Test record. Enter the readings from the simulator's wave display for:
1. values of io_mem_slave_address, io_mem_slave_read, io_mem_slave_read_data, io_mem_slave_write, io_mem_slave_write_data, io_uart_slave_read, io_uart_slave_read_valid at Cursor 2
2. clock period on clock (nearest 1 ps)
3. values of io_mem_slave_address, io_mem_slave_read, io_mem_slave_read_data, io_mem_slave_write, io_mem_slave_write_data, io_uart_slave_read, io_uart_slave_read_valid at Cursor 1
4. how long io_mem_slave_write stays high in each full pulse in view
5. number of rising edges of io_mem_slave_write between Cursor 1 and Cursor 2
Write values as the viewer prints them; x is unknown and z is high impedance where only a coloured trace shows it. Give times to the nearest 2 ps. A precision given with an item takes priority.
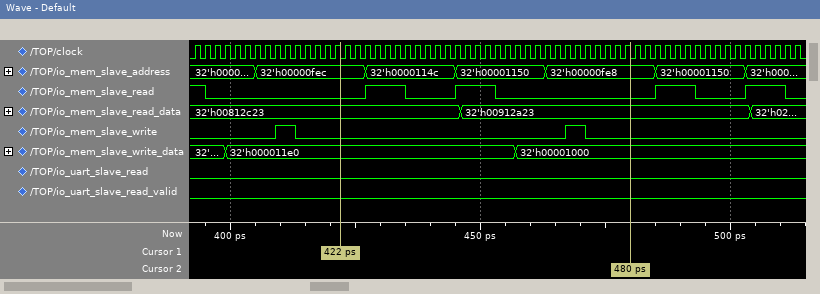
io_mem_slave_address=32'h00000fe8, io_mem_slave_read=0, io_mem_slave_read_data=32'h00912a23, io_mem_slave_write=0, io_mem_slave_write_data=32'h00001000, io_uart_slave_read=0, io_uart_slave_read_valid=0
2 ps
io_mem_slave_address=32'h00000fec, io_mem_slave_read=0, io_mem_slave_read_data=32'h00812c23, io_mem_slave_write=0, io_mem_slave_write_data=32'h000011e0, io_uart_slave_read=0, io_uart_slave_read_valid=0
4 ps, 4 ps
1
